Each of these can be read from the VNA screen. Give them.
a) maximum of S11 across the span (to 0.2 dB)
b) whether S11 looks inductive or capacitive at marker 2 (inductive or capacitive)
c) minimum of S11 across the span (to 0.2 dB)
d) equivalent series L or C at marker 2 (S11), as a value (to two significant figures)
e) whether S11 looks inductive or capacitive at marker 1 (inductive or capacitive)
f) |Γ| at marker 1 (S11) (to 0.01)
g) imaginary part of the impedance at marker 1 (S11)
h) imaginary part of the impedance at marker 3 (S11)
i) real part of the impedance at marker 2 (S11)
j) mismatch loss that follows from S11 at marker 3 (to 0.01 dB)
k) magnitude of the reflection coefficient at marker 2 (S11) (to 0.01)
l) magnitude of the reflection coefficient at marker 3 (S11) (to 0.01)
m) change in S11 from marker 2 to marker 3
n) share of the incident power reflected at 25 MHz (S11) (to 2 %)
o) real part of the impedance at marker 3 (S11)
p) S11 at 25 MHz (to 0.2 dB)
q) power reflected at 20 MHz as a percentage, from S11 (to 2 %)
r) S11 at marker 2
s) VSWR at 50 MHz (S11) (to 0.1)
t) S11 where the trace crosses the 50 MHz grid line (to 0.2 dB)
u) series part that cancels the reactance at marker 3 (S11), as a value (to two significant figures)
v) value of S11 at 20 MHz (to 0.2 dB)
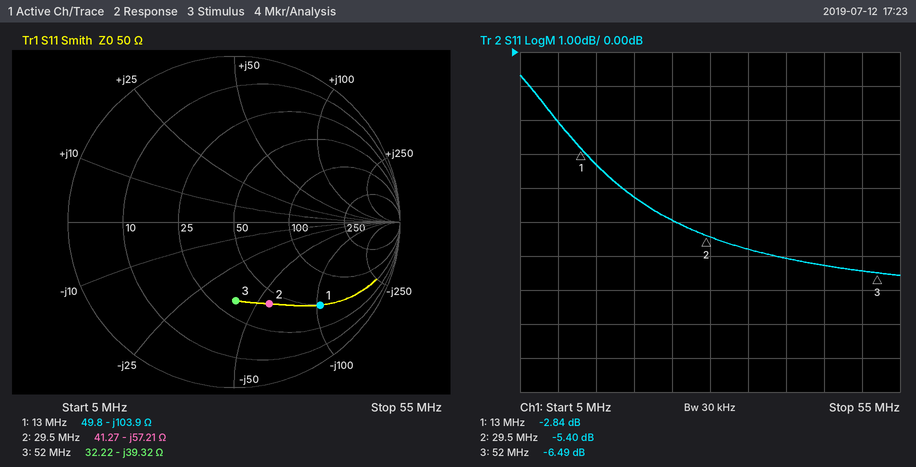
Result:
-0.6 dB
capacitive
-6.6 dB
94 pF
capacitive
0.72
-103.9 Ω
-39.32 Ω
41.27 Ω
1.10 dB
0.54
0.47
-1.09 dB
32 %
32.22 Ω
-5.0 dB
38 %
-5.40 dB
2.8
-6.4 dB
120 nH
-4.2 dB
